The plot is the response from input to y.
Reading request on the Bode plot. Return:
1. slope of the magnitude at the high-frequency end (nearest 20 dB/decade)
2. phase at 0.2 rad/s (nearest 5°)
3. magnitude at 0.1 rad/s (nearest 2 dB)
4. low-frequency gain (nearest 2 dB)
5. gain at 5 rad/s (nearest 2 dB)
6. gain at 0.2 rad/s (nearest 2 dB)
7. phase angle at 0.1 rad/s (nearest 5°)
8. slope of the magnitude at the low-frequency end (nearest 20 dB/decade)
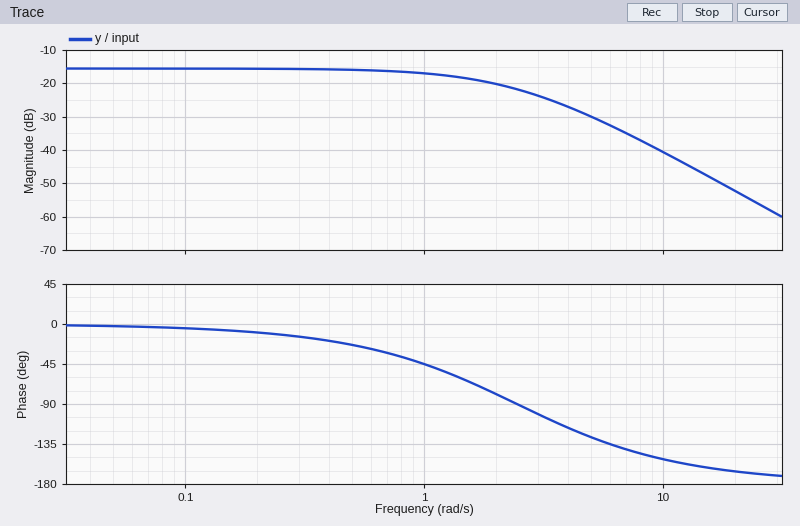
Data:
-40 dB/decade
-10°
-16 dB
-16 dB
-30 dB
-16 dB
-5°
0 dB/decade
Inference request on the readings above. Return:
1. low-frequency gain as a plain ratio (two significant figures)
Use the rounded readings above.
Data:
0.16
